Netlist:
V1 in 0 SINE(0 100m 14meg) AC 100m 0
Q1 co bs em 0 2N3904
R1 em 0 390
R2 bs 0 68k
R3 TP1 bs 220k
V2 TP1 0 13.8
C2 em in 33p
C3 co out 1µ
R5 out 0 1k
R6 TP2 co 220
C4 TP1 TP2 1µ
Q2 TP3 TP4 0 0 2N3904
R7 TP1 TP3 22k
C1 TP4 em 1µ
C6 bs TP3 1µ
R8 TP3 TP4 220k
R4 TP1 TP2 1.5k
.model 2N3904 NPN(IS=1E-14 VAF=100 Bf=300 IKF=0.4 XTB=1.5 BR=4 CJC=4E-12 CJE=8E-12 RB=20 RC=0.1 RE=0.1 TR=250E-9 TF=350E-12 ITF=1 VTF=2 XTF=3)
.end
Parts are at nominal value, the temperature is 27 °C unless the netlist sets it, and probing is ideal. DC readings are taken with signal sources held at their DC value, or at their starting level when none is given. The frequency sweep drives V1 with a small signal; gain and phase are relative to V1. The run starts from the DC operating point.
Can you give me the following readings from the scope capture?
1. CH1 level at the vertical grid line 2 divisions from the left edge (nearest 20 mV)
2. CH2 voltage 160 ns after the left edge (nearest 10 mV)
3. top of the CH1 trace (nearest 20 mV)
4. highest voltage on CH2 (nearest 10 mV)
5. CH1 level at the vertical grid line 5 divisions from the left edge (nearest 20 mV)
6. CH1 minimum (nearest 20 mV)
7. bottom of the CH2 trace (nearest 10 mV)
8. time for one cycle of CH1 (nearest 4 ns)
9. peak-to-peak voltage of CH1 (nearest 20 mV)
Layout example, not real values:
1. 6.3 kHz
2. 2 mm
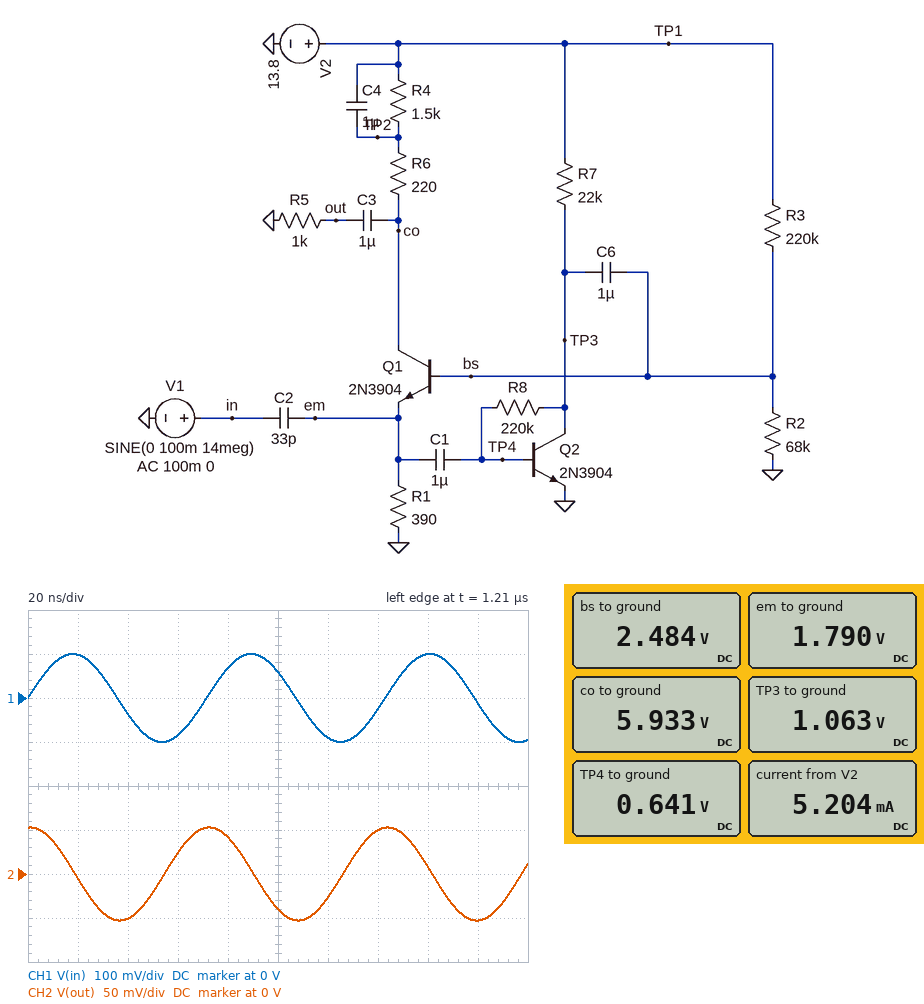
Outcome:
1. -40 mV
2. 10 mV
3. 100 mV
4. 50 mV
5. 60 mV
6. -100 mV
7. -50 mV
8. 72 ns
9. 200 mV
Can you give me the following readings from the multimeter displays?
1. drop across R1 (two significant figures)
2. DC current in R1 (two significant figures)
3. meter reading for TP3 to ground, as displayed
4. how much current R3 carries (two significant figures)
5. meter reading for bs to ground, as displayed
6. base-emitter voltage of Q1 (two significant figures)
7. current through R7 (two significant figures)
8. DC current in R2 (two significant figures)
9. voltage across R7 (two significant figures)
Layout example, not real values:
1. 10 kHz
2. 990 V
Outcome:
1. 1.8 V
2. 4.6 mA
3. 1.063 V
4. 51 µA
5. 2.484 V
6. 690 mV
7. 580 µA
8. 37 µA
9. 13 V
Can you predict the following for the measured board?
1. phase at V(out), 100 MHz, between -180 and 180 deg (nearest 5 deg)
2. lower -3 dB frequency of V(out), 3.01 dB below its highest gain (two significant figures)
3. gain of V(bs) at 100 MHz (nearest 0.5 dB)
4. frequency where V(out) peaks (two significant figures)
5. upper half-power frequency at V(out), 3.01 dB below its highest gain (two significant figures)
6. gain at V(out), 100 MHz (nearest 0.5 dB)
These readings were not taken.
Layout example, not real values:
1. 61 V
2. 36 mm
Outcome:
1. 5 deg
2. 88 MHz
3. 0.5 dB
4. 110 MHz
5. 130 MHz
6. 19.0 dB
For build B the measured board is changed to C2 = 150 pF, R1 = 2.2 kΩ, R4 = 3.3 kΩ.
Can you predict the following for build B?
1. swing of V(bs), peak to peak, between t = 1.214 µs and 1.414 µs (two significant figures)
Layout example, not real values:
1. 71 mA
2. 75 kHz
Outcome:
1. 240 mV
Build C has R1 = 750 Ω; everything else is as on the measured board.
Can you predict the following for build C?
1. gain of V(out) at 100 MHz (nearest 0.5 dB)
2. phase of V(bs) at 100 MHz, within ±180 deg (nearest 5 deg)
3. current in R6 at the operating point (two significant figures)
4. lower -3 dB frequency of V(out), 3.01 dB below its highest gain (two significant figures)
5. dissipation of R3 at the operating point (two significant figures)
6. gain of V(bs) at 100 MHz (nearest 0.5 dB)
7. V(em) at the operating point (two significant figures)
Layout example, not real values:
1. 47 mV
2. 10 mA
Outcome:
1. 20.0 dB
2. 155 deg
3. 2.8 mA
4. 90 MHz
5. 550 µW
6. 2.0 dB
7. 2.1 V
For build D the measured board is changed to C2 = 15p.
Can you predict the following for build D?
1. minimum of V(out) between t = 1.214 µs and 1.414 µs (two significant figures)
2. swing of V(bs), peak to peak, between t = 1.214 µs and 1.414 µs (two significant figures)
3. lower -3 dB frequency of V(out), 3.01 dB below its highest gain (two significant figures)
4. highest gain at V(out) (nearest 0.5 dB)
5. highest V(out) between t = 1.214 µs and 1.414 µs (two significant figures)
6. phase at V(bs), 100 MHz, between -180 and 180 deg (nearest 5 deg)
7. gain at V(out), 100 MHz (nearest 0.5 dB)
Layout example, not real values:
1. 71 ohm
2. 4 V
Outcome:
1. -24 mV
2. 1.6 mV
3. 96 MHz
4. 11.0 dB
5. 24 mV
6. 170 deg
7. 9.0 dB
